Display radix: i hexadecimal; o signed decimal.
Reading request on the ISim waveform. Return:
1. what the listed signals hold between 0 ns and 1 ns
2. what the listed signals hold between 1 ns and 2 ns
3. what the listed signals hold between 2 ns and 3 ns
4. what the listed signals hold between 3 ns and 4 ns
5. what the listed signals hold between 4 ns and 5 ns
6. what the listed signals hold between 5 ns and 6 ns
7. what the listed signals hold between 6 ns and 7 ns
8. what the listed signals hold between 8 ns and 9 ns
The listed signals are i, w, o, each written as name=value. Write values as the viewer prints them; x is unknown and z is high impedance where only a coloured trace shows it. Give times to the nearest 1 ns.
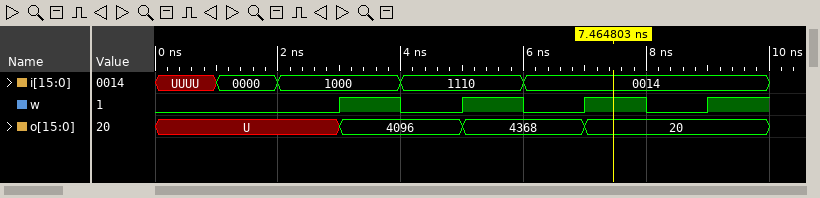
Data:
i=UUUU, w=0, o=U
i=0000, w=0, o=U
i=1000, w=0, o=U
i=1000, w=1, o=4096
i=1110, w=0, o=4096
i=1110, w=1, o=4368
i=0014, w=0, o=4368
i=0014, w=0, o=20
